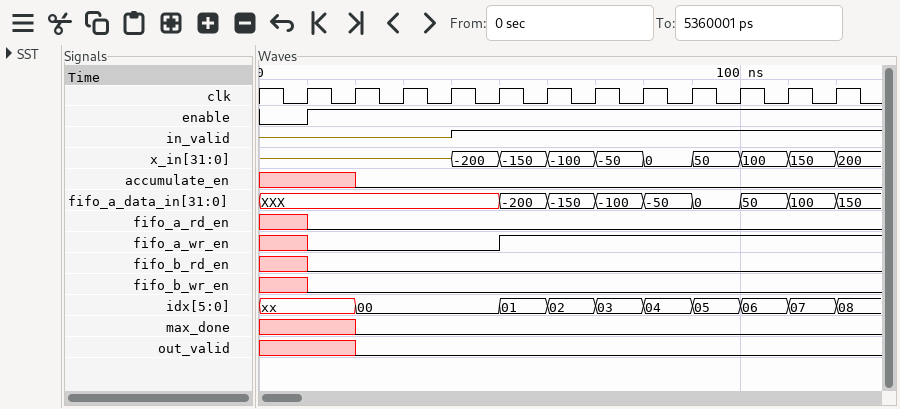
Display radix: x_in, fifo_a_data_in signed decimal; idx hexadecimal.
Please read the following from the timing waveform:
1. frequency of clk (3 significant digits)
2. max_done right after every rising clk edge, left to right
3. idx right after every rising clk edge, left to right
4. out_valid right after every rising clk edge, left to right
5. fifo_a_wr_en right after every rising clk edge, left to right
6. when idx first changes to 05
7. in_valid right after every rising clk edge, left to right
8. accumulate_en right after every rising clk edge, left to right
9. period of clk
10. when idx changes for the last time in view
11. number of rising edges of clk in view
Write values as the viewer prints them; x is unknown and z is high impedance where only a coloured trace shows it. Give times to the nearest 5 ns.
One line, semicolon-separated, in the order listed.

100 MHz; x 0 0 0 0 0 0 0 0 0 0 0; xx, 00, 00, 00, 01, 02, 03, 04, 05, 06, 07, 08; x 0 0 0 0 0 0 0 0 0 0 0; 0 0 0 0 1 1 1 1 1 1 1 1; 90 ns; z z z 1 1 1 1 1 1 1 1 1; x 0 0 0 0 0 0 0 0 0 0 0; 10 ns; 120 ns; 12
